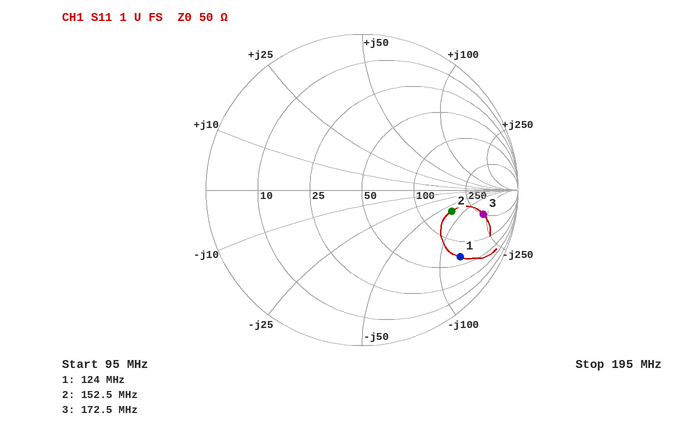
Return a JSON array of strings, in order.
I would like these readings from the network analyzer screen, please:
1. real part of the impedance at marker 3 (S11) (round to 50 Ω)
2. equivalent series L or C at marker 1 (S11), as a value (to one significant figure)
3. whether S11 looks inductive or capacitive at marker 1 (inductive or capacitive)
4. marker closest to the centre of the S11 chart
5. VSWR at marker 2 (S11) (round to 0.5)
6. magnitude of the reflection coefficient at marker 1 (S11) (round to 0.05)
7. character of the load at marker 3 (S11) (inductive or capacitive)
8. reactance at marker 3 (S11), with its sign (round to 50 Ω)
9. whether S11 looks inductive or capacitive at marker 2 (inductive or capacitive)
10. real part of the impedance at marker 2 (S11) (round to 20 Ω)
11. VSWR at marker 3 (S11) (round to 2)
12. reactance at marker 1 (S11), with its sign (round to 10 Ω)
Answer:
["250 Ω", "10 pF", "capacitive", "marker 2", "4.0", "0.75", "capacitive", "-200 Ω", "capacitive", "160 Ω", "8", "-130 Ω"]
